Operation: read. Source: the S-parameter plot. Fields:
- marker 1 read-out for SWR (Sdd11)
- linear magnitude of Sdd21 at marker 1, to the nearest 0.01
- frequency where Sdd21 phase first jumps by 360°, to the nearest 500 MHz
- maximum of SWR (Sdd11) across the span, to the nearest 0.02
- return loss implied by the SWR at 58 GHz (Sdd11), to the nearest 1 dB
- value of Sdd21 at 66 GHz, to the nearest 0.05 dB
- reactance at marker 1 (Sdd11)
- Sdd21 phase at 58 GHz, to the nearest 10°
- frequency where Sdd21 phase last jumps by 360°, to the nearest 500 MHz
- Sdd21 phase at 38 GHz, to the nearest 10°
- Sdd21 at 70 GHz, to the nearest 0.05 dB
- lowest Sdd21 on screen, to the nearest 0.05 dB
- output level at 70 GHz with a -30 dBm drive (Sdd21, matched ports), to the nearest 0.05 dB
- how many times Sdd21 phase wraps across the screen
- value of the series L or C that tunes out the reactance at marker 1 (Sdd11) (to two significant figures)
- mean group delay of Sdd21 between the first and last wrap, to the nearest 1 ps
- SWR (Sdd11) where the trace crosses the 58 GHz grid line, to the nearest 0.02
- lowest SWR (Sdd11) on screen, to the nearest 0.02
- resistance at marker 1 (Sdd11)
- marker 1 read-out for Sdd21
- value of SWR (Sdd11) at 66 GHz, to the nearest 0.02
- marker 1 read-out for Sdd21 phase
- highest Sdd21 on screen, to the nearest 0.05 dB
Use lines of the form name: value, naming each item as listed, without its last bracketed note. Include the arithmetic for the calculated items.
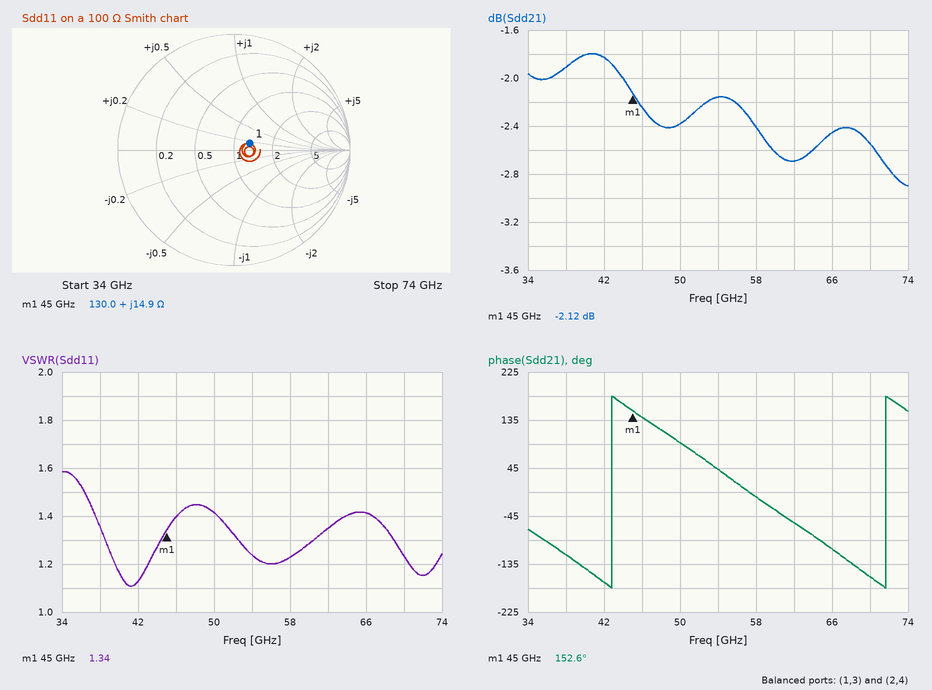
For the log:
marker 1 read-out for SWR: 1.34
linear magnitude of Sdd21 at marker 1, to the nearest 0.01: 10^(-2.12/20) ≈ 0.78
frequency where Sdd21 phase first jumps by 360°, to the nearest 500 MHz: 43.0 GHz
maximum of SWR (Sdd11) across the span, to the nearest 0.02: 1.58
return loss implied by the SWR at 58 GHz (Sdd11), to the nearest 1 dB: −20 log10((1.22 − 1)/(1.22 + 1)) ≈ 20 dB
value of Sdd21 at 66 GHz, to the nearest 0.05 dB: -2.45 dB
reactance at marker 1: +14.9 Ω
Sdd21 phase at 58 GHz, to the nearest 10°: -10°
frequency where Sdd21 phase last jumps by 360°, to the nearest 500 MHz: 71.5 GHz
Sdd21 phase at 38 GHz, to the nearest 10°: -120°
Sdd21 at 70 GHz, to the nearest 0.05 dB: -2.55 dB
lowest Sdd21 on screen, to the nearest 0.05 dB: -2.90 dB
output level at 70 GHz with a -30 dBm drive (Sdd21, matched ports), to the nearest 0.05 dB: -30 dBm + (-2.55 dB) = -32.55 dBm
how many times Sdd21 phase wraps across the screen: 2
value of the series L or C that tunes out the reactance at marker 1 (Sdd11): C = 1/(2π × 45 GHz × 14.9 Ω) ≈ 237 fF, so 240 fF to two significant figures
mean group delay of Sdd21 between the first and last wrap, to the nearest 1 ps: 1 cycle / (71.5 GHz − 43.0 GHz) ≈ 35 ps
SWR (Sdd11) where the trace crosses the 58 GHz grid line, to the nearest 0.02: 1.22
lowest SWR (Sdd11) on screen, to the nearest 0.02: 1.10
resistance at marker 1: 130.0 Ω
marker 1 read-out for Sdd21: -2.12 dB
value of SWR (Sdd11) at 66 GHz, to the nearest 0.02: 1.42
marker 1 read-out for Sdd21 phase: 152.6°
highest Sdd21 on screen, to the nearest 0.05 dB: -1.80 dB
